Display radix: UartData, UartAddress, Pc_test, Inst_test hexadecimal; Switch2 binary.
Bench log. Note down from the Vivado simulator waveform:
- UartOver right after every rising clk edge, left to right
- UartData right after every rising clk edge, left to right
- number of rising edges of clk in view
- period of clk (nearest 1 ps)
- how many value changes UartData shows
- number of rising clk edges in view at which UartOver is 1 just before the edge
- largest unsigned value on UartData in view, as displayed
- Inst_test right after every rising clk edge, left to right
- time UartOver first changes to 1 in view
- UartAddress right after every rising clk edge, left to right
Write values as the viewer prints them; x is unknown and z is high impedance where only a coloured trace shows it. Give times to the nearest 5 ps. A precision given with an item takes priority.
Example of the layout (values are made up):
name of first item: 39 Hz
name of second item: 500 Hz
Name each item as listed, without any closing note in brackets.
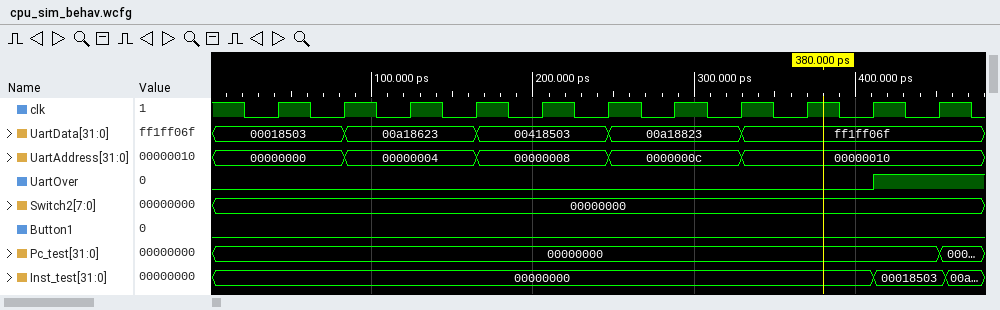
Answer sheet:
UartOver right after every rising clk edge, left to right: 0 0 0 0 0 0 0 0 0 1 1
UartData right after every rising clk edge, left to right: 00018503, 00a18623, 00a18623, 00418503, 00418503, 00a18823, 00a18823, ff1ff06f, ff1ff06f, ff1ff06f, ff1ff06f
number of rising edges of clk in view: 11
period of clk: 41 ps
how many value changes UartData shows: 4
number of rising clk edges in view at which UartOver is 1 just before the edge: 1
largest unsigned value on UartData in view, as displayed: ff1ff06f
Inst_test right after every rising clk edge, left to right: 00000000, 00000000, 00000000, 00000000, 00000000, 00000000, 00000000, 00000000, 00000000, 00018503, 00018503
time UartOver first changes to 1 in view: 410 ps
UartAddress right after every rising clk edge, left to right: 00000000, 00000004, 00000004, 00000008, 00000008, 0000000c, 0000000c, 00000010, 00000010, 00000010, 00000010
